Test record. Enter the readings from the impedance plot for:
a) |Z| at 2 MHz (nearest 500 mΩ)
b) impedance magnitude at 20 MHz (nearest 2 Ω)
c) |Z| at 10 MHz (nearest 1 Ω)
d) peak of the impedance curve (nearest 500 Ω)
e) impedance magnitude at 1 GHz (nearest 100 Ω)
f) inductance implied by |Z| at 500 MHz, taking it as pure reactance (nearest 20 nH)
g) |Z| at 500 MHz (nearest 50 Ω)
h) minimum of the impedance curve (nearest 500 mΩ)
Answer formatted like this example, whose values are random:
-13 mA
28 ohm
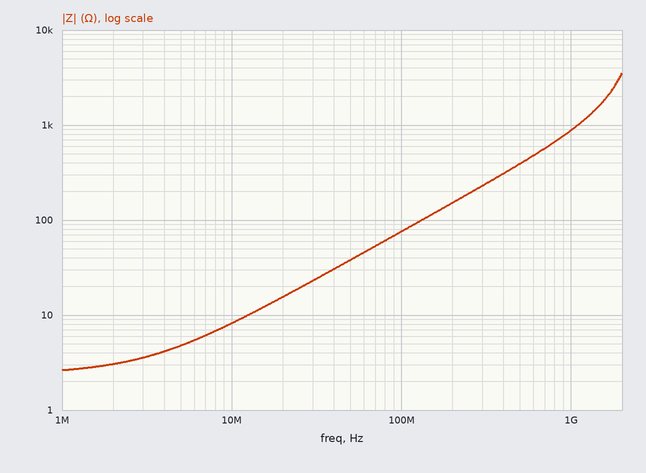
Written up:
3.0 Ω
16 Ω
8 Ω
3.5 kΩ
900 Ω
120 nH
400 Ω
2.5 Ω
